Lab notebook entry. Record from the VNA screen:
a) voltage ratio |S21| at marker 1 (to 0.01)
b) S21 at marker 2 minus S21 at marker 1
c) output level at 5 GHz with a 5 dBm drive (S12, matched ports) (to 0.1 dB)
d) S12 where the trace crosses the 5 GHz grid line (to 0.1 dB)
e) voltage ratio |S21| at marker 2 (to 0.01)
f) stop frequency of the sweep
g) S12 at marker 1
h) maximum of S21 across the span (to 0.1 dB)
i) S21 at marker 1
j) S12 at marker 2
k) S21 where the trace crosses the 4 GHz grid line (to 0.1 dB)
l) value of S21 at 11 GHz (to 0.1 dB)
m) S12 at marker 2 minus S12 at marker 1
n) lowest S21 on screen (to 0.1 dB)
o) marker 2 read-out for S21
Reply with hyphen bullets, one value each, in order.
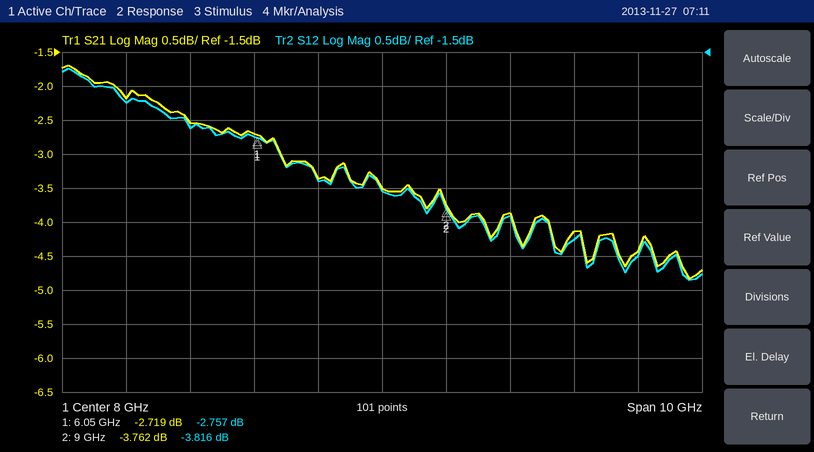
- 0.73
- -1.043 dB
- 2.4 dBm
- -2.6 dB
- 0.65
- 13 GHz
- -2.757 dB
- -1.7 dB
- -2.719 dB
- -3.816 dB
- -2.2 dB
- -4.1 dB
- -1.059 dB
- -4.8 dB
- -3.762 dB
